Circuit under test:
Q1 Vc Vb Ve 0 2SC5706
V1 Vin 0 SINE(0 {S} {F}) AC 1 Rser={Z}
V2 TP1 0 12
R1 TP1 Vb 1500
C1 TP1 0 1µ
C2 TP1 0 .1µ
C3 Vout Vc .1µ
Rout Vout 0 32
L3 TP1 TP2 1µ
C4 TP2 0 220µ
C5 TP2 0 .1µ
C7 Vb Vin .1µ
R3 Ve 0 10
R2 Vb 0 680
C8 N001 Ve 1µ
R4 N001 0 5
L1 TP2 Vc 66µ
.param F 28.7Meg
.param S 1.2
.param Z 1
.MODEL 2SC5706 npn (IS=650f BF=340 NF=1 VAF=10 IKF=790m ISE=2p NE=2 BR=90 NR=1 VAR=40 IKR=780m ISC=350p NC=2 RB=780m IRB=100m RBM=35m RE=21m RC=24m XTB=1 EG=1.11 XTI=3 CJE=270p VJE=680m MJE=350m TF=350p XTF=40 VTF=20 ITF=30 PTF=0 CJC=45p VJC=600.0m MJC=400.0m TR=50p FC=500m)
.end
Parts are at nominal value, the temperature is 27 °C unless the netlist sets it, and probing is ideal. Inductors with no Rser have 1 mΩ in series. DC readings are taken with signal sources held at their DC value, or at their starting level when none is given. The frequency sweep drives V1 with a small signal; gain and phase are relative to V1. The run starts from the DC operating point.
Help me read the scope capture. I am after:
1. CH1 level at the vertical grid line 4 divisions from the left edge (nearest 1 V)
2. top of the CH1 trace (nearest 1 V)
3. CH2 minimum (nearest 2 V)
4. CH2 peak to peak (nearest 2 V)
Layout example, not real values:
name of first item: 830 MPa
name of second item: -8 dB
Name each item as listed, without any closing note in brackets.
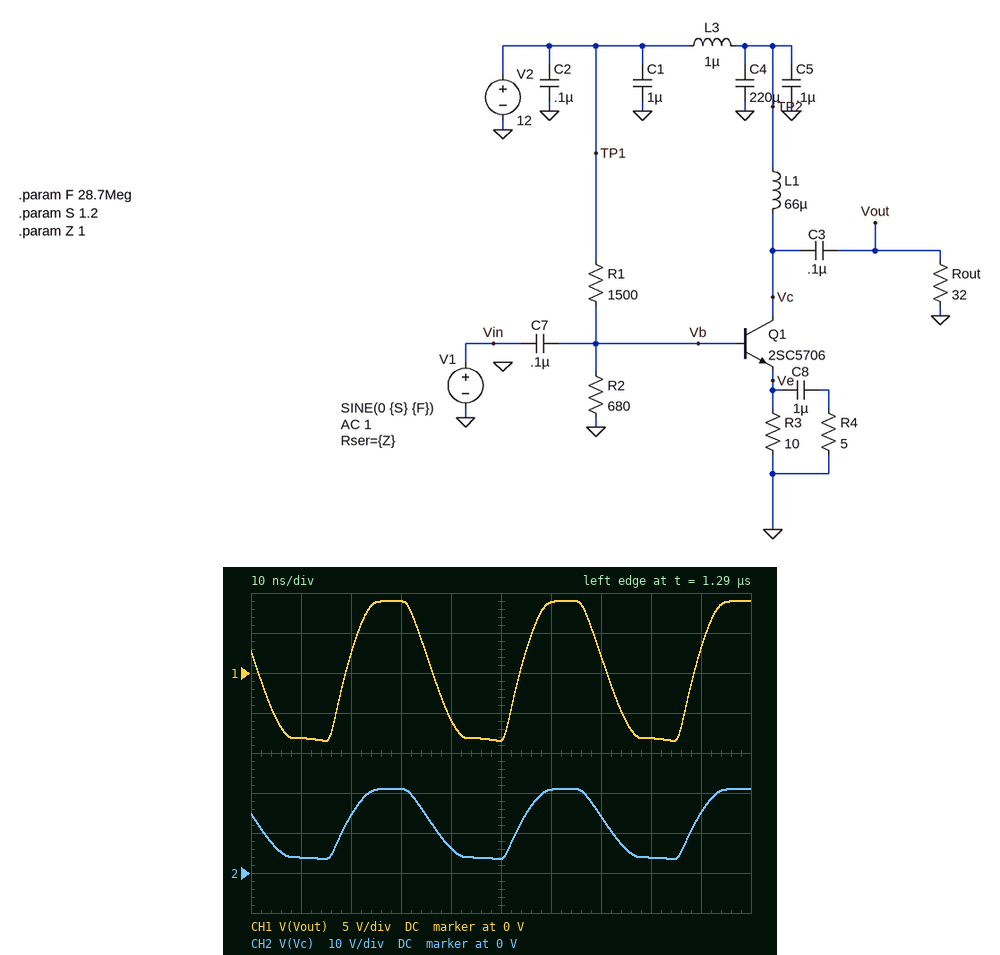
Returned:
CH1 level at the vertical grid line 4 divisions from the left edge: -6 V
top of the CH1 trace: 9 V
CH2 minimum: 4 V
CH2 peak to peak: 18 V
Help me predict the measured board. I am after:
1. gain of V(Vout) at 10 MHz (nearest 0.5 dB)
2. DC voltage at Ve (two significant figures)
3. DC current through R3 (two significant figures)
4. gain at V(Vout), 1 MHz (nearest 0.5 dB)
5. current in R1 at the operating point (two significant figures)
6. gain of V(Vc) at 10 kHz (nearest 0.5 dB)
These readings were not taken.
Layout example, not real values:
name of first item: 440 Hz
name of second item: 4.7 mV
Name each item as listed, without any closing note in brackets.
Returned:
gain of V(Vout) at 10 MHz: 19.0 dB
DC voltage at Ve: 2.8 V
DC current through R3: 280 mA
gain at V(Vout), 1 MHz: 19.0 dB
current in R1 at the operating point: 5.7 mA
gain of V(Vc) at 10 kHz: -5.0 dB
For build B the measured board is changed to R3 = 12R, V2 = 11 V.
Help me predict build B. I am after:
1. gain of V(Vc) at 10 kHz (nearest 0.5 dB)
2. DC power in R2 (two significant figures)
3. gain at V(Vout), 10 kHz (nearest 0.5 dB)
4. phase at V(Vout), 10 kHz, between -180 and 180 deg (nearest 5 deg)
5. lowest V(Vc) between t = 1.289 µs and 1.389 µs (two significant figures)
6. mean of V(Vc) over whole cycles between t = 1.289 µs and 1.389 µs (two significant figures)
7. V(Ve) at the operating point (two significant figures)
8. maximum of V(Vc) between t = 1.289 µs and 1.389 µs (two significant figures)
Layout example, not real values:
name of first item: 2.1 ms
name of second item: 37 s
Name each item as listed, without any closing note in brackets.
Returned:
gain of V(Vc) at 10 kHz: -6.0 dB
DC power in R2: 15 mW
gain at V(Vout), 10 kHz: -20.0 dB
phase at V(Vout), 10 kHz, between -180 and 180 deg: 35 deg
lowest V(Vc) between t = 1.289 µs and 1.389 µs: 3.2 V
mean of V(Vc) over whole cycles between t = 1.289 µs and 1.389 µs: 11 V
V(Ve) at the operating point: 2.6 V
maximum of V(Vc) between t = 1.289 µs and 1.389 µs: 18 V
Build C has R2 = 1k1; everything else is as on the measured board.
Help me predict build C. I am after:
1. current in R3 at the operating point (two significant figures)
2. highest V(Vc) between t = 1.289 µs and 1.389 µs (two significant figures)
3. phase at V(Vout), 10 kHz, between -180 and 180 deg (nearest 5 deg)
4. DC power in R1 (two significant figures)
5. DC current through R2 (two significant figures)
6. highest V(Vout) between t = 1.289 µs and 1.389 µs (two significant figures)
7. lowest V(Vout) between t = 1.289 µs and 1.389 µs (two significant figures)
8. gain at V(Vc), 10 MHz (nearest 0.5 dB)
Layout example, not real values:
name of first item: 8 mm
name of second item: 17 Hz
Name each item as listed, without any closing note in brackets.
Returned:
current in R3 at the operating point: 380 mA
highest V(Vc) between t = 1.289 µs and 1.389 µs: 23 V
phase at V(Vout), 10 kHz, between -180 and 180 deg: 30 deg
DC power in R1: 37 mW
DC current through R2: 4.1 mA
highest V(Vout) between t = 1.289 µs and 1.389 µs: 11 V
lowest V(Vout) between t = 1.289 µs and 1.389 µs: -7.8 V
gain at V(Vc), 10 MHz: 19.0 dB
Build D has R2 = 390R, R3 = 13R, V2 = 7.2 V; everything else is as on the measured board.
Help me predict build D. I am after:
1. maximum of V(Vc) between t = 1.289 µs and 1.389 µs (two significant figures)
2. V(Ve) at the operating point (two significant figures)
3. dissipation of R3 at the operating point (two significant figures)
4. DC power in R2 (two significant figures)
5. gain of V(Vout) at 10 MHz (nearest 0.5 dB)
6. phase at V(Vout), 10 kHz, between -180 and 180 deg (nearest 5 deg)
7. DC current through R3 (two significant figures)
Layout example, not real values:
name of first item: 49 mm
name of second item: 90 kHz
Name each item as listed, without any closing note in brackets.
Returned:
maximum of V(Vc) between t = 1.289 µs and 1.389 µs: 9.7 V
V(Ve) at the operating point: 800 mV
dissipation of R3 at the operating point: 50 mW
DC power in R2: 5.4 mW
gain of V(Vout) at 10 MHz: 17.5 dB
phase at V(Vout), 10 kHz, between -180 and 180 deg: 45 deg
DC current through R3: 62 mA
